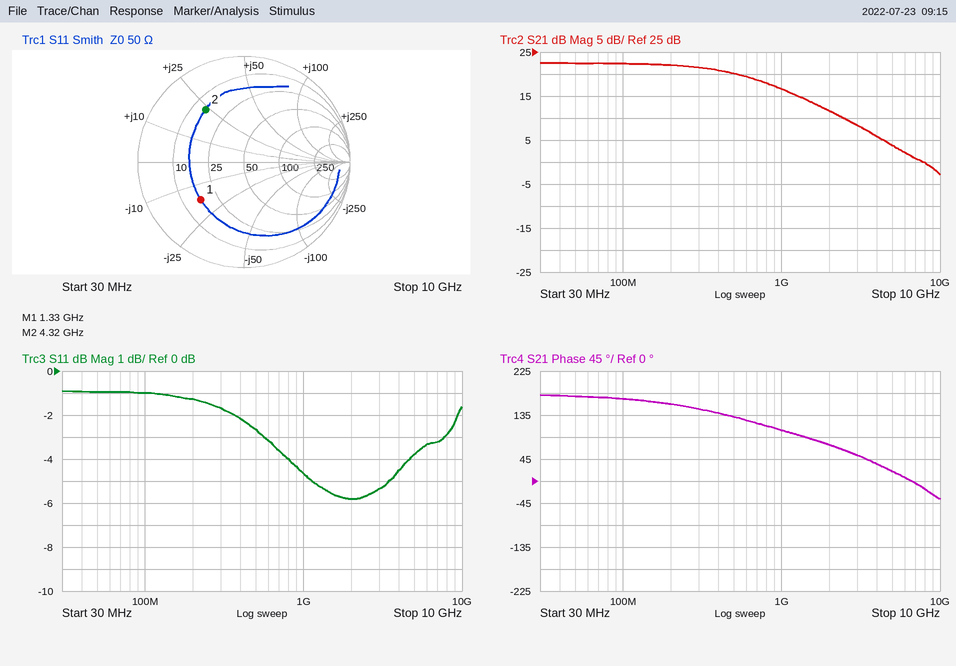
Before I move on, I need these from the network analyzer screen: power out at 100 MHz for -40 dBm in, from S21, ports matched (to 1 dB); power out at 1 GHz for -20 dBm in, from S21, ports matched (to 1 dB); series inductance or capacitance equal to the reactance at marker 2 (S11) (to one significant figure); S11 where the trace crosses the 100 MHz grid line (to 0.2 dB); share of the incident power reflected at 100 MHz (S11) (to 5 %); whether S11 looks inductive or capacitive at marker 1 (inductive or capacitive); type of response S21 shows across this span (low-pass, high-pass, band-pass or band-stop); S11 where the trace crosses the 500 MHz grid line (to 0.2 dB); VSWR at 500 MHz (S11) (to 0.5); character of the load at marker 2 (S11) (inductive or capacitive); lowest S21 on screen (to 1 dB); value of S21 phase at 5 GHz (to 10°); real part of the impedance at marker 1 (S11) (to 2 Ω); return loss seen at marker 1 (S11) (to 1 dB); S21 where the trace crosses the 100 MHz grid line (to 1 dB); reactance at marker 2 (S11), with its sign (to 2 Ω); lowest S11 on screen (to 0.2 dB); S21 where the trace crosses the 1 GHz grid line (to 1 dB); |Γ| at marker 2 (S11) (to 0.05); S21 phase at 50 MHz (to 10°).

-18 dBm
-3 dBm
900 pH
-1.0 dB
80 %
capacitive
low-pass
-2.6 dB
6.5
inductive
-3 dB
20°
16 Ω
5 dB
22 dB
+24 Ω
-5.8 dB
17 dB
0.60
170°
